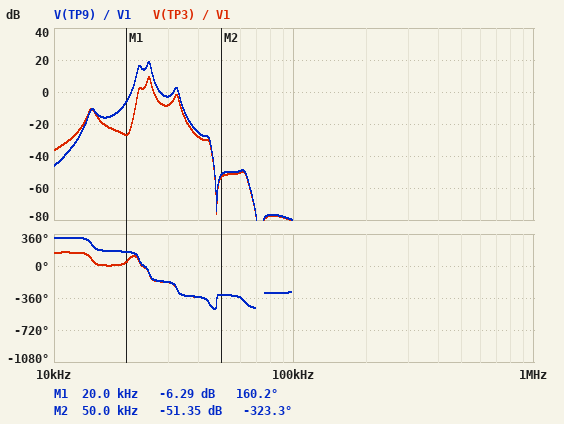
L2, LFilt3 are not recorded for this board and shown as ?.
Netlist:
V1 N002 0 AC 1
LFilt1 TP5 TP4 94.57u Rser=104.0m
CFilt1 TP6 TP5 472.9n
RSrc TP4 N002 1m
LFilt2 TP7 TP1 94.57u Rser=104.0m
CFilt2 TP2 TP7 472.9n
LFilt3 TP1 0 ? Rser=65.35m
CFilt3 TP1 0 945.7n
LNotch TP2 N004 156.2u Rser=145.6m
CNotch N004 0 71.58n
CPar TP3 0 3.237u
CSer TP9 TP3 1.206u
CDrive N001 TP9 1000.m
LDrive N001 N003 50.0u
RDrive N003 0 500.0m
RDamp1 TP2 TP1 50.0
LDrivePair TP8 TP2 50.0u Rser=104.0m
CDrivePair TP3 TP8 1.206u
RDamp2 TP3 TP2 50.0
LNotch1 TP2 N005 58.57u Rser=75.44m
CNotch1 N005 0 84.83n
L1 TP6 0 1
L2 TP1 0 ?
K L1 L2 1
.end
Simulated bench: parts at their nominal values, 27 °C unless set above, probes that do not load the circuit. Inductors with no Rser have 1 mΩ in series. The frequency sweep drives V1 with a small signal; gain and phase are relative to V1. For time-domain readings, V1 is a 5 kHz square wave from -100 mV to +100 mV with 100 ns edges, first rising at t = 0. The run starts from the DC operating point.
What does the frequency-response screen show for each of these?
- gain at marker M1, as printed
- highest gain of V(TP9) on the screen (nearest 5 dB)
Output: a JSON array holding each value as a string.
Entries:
["-6.29 dB", "20 dB"]
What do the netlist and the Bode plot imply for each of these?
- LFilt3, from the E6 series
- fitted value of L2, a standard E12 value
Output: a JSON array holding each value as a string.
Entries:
["68 µH", "2.2 H"]
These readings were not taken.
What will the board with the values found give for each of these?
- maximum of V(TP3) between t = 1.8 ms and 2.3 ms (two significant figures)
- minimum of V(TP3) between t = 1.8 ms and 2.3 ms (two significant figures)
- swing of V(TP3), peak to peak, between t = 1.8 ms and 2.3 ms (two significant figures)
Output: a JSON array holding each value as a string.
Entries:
["79 mV", "-79 mV", "160 mV"]
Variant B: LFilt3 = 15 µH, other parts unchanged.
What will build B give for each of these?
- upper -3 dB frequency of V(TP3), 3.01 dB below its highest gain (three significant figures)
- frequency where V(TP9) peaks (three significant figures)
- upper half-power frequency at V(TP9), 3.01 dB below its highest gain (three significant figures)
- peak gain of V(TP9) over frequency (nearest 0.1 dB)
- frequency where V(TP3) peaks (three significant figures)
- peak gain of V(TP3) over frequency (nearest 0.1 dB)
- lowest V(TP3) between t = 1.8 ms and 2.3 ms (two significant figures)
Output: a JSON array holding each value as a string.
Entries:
["23.4 kHz", "23.0 kHz", "23.3 kHz", "21.6 dB", "23.1 kHz", "8.4 dB", "-42 mV"]
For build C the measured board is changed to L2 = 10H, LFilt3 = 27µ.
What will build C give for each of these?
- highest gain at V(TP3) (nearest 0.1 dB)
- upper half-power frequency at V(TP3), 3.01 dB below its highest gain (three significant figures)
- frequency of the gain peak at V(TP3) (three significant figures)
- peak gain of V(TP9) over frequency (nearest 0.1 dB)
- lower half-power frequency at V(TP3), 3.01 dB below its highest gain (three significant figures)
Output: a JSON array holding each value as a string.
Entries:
["10.3 dB", "24.1 kHz", "23.5 kHz", "22.5 dB", "23.2 kHz"]
